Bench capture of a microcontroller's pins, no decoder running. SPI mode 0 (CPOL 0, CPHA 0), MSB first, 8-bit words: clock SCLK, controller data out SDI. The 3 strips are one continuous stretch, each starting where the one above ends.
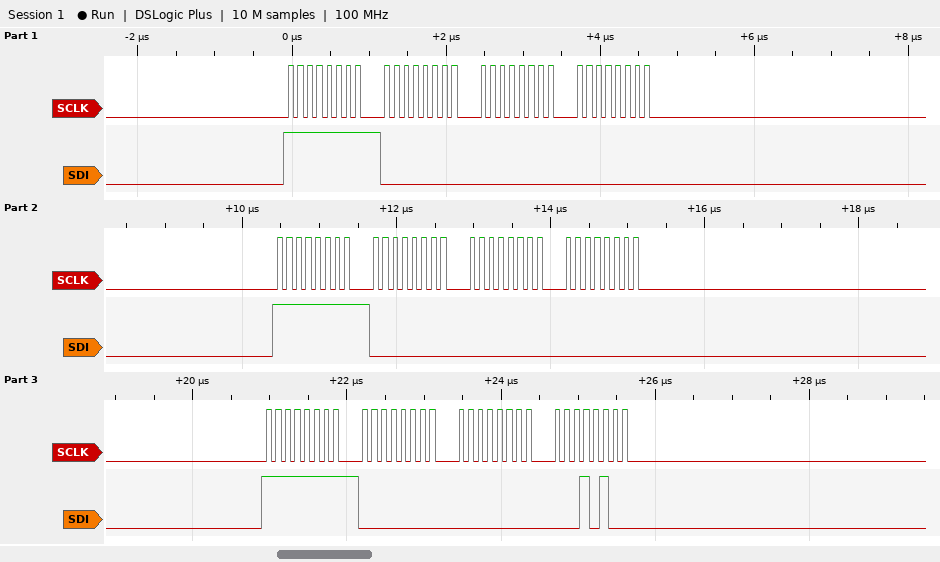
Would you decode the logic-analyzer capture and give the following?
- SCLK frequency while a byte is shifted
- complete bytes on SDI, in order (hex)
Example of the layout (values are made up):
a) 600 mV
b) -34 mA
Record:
a) 8 MHz
b) FF 00 00 00 FF 00 00 00 FF 00 00 14
